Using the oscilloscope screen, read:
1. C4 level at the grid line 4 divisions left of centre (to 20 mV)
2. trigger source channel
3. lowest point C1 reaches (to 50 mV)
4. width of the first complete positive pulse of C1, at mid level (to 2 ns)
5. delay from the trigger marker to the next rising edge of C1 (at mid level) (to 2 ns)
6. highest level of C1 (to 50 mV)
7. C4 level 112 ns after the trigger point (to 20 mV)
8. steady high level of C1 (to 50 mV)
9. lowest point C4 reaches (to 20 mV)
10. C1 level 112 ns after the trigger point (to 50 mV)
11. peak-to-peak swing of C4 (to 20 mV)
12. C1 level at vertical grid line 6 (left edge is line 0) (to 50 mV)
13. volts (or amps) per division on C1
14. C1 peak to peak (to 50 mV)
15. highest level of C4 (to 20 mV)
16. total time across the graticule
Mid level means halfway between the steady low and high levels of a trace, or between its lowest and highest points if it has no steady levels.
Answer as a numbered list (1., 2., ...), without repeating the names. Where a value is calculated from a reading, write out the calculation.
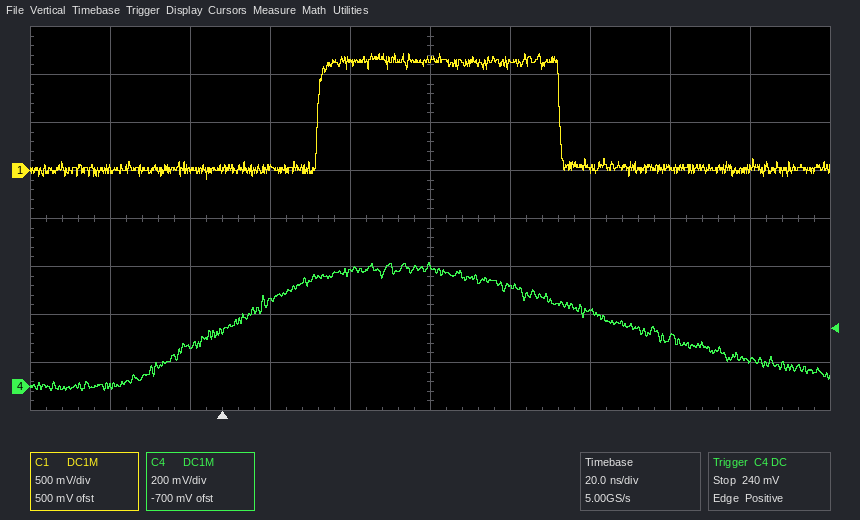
1. 0 mV
2. C4
3. -100 mV
4. 60 ns
5. 24 ns
6. 1.20 V
7. 200 mV
8. 1.15 V
9. -20 mV
10. 50 mV
11. 520 mV − (-20 mV) = 540 mV
12. 1.10 V
13. 500 mV
14. 1.20 V − (-100 mV) = 1.30 V
15. 520 mV
16. 200 ns
